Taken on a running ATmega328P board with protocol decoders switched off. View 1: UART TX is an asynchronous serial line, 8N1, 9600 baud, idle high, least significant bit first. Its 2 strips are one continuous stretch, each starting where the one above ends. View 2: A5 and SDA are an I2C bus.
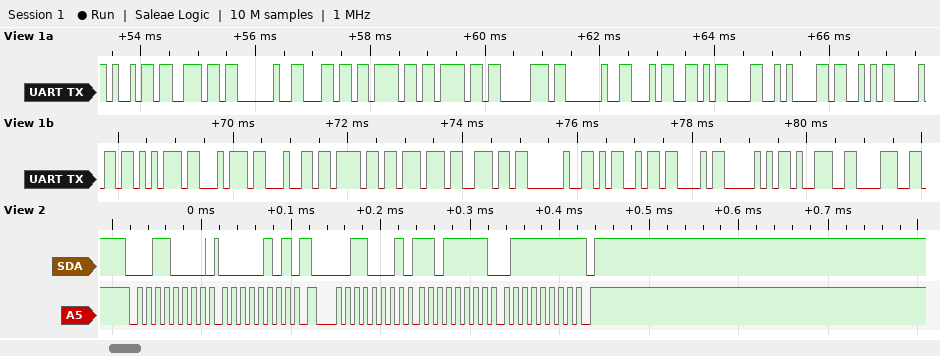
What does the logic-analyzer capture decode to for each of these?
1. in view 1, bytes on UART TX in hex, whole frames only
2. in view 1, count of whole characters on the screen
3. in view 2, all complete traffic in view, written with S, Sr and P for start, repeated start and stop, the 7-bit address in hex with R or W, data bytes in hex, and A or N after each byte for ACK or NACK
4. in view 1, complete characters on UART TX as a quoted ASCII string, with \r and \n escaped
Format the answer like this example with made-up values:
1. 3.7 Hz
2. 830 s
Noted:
1. 69 6E 20 6C 6F 6F 70 20 34 0D 0A 53 68 75 74 64 6F 77 6E 20 4D 43 50 39 38
2. 25
3. S 18W A 05 A Sr 18R A DF A 7F N P
4. "in loop 4\r\nShutdown MCP98"
